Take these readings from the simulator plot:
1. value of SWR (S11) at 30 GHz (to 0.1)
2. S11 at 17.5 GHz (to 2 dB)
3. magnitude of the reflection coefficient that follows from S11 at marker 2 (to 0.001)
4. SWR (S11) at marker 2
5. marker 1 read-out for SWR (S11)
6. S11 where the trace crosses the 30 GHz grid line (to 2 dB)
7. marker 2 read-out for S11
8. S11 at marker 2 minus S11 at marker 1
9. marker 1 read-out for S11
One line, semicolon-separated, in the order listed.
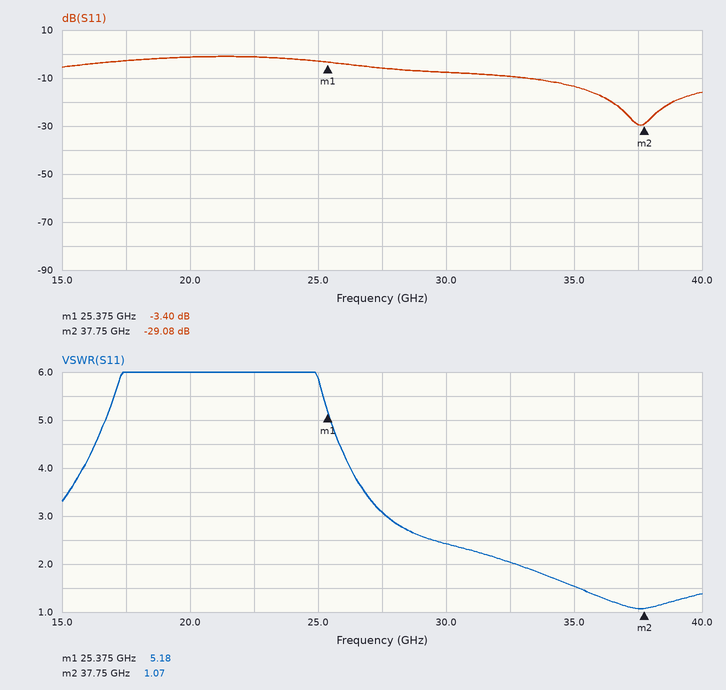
2.4; -2 dB; 0.035; 1.07; 5.18; -8 dB; -29.08 dB; -25.68 dB; -3.40 dB
